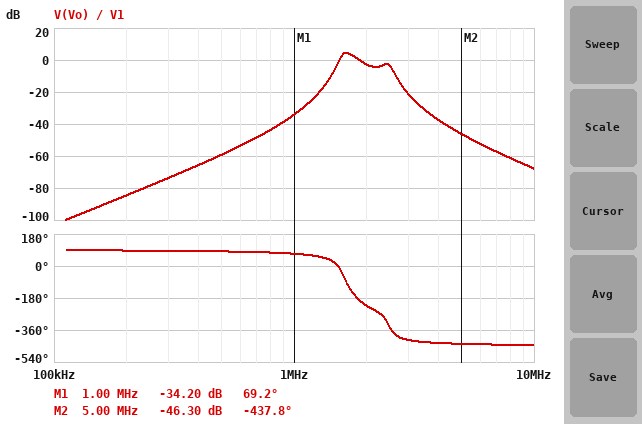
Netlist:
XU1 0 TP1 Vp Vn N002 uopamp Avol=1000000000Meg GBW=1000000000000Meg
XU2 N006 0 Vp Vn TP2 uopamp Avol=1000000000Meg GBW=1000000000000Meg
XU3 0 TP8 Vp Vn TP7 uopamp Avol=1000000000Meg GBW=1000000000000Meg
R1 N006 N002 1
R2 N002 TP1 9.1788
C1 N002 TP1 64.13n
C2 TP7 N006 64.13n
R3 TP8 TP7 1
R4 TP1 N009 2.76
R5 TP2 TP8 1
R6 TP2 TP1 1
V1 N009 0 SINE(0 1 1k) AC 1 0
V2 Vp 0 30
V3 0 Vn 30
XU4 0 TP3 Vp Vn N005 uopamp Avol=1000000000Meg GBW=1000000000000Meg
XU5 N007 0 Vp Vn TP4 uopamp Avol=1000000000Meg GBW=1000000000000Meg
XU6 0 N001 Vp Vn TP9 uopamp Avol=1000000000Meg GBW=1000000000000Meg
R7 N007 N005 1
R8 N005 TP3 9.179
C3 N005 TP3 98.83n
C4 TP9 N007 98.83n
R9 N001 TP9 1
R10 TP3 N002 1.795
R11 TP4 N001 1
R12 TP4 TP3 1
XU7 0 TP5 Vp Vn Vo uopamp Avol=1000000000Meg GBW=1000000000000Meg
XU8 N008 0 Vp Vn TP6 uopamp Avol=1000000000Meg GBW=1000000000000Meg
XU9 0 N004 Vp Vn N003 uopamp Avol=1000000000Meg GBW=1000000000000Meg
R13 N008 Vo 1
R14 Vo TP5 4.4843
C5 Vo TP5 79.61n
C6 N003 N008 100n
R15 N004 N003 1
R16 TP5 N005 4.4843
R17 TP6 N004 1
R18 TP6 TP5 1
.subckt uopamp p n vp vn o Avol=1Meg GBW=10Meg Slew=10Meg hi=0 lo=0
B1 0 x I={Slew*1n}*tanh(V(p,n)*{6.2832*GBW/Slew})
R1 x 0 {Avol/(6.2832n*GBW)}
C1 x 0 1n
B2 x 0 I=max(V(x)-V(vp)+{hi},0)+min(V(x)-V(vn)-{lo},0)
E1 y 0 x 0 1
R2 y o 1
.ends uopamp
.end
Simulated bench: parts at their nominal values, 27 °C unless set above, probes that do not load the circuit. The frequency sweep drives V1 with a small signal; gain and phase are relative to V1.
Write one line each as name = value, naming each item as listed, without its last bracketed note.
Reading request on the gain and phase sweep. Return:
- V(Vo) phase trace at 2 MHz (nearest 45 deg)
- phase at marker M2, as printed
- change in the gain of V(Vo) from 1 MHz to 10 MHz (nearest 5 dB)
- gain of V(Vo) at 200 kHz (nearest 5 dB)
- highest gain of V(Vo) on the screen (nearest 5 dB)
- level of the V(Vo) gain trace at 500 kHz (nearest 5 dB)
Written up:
V(Vo) phase trace at 2 MHz = -225 deg
phase at marker M2, as printed = -437.8 deg
change in the gain of V(Vo) from 1 MHz to 10 MHz = -35 dB
gain of V(Vo) at 200 kHz = -85 dB
highest gain of V(Vo) on the screen = 5 dB
level of the V(Vo) gain trace at 500 kHz = -60 dB
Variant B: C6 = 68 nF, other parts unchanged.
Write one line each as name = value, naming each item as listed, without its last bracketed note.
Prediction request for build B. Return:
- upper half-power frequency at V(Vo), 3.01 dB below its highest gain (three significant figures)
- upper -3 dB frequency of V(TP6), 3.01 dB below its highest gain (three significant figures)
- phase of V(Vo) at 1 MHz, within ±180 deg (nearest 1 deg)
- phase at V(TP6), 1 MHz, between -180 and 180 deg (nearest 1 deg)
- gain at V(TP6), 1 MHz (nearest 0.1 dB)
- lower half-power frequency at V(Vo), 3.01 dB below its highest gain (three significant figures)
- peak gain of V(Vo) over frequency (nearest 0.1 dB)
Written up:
upper half-power frequency at V(Vo), 3.01 dB below its highest gain = 2.54 MHz
upper -3 dB frequency of V(TP6), 3.01 dB below its highest gain = 2.53 MHz
phase of V(Vo) at 1 MHz, within ±180 deg = 74 deg
phase at V(TP6), 1 MHz, between -180 and 180 deg = -16 deg
gain at V(TP6), 1 MHz = -31.2 dB
lower half-power frequency at V(Vo), 3.01 dB below its highest gain = 2.08 MHz
peak gain of V(Vo) over frequency = 2.6 dB
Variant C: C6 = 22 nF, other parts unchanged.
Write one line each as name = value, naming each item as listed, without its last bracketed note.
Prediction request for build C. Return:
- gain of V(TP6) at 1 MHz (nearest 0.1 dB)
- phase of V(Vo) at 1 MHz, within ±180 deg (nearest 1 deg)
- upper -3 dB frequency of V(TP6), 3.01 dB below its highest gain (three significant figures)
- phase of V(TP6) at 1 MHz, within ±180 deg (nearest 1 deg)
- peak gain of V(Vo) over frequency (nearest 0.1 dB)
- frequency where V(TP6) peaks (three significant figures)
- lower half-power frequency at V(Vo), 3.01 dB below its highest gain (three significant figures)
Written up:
gain of V(TP6) at 1 MHz = -32.6 dB
phase of V(Vo) at 1 MHz, within ±180 deg = 79 deg
upper -3 dB frequency of V(TP6), 3.01 dB below its highest gain = 2.61 MHz
phase of V(TP6) at 1 MHz, within ±180 deg = -11 deg
peak gain of V(Vo) over frequency = -11.3 dB
frequency where V(TP6) peaks = 2.47 MHz
lower half-power frequency at V(Vo), 3.01 dB below its highest gain = 2.35 MHz
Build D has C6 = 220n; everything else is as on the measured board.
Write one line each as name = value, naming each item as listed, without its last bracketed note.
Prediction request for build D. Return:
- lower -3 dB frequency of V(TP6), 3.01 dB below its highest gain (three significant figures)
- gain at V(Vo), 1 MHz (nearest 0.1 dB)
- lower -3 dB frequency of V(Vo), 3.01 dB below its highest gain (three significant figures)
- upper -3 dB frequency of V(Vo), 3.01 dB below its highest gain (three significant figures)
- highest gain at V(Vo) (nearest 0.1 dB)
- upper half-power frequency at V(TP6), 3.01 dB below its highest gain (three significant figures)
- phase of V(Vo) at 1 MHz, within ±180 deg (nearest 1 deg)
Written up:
lower -3 dB frequency of V(TP6), 3.01 dB below its highest gain = 1.51 MHz
gain at V(Vo), 1 MHz = -23.2 dB
lower -3 dB frequency of V(Vo), 3.01 dB below its highest gain = 1.52 MHz
upper -3 dB frequency of V(Vo), 3.01 dB below its highest gain = 1.70 MHz
highest gain at V(Vo) = 0.8 dB
upper half-power frequency at V(TP6), 3.01 dB below its highest gain = 1.69 MHz
phase of V(Vo) at 1 MHz, within ±180 deg = 36 deg
